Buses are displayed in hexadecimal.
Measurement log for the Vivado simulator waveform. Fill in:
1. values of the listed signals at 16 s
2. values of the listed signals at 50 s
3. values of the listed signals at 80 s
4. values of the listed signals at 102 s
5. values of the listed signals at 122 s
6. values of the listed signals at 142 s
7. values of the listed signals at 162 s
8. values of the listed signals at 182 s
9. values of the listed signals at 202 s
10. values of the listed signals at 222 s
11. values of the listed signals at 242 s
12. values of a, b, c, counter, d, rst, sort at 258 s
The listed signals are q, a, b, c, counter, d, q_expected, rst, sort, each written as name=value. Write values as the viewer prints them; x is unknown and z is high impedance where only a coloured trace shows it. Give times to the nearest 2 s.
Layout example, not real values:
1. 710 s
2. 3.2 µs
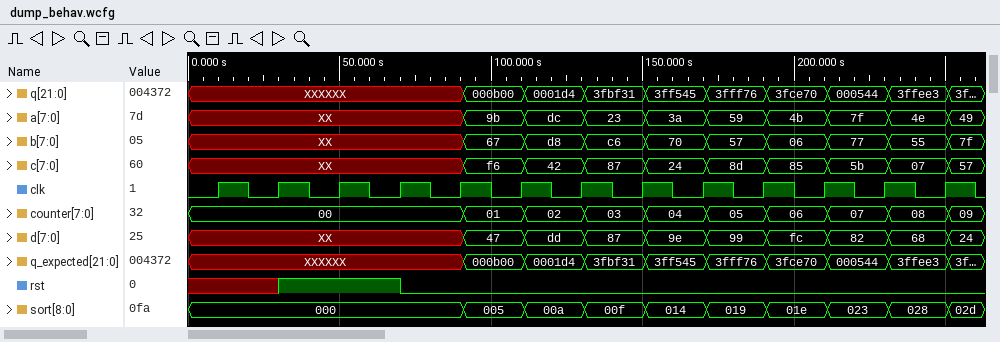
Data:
1. q=XXXXXX, a=XX, b=XX, c=XX, counter=00, d=XX, q_expected=XXXXXX, rst=x, sort=000
2. q=XXXXXX, a=XX, b=XX, c=XX, counter=00, d=XX, q_expected=XXXXXX, rst=1, sort=000
3. q=XXXXXX, a=XX, b=XX, c=XX, counter=00, d=XX, q_expected=XXXXXX, rst=0, sort=000
4. q=000b00, a=9b, b=67, c=f6, counter=01, d=47, q_expected=000b00, rst=0, sort=005
5. q=0001d4, a=dc, b=d8, c=42, counter=02, d=dd, q_expected=0001d4, rst=0, sort=00a
6. q=3fbf31, a=23, b=c6, c=87, counter=03, d=87, q_expected=3fbf31, rst=0, sort=00f
7. q=3ff545, a=3a, b=70, c=24, counter=04, d=9e, q_expected=3ff545, rst=0, sort=014
8. q=3fff76, a=59, b=57, c=8d, counter=05, d=99, q_expected=3fff76, rst=0, sort=019
9. q=3fce70, a=4b, b=06, c=85, counter=06, d=fc, q_expected=3fce70, rst=0, sort=01e
10. q=000544, a=7f, b=77, c=5b, counter=07, d=82, q_expected=000544, rst=0, sort=023
11. q=3ffee3, a=4e, b=55, c=07, counter=08, d=68, q_expected=3ffee3, rst=0, sort=028
12. a=49, b=7f, c=57, counter=09, d=24, rst=0, sort=02d
